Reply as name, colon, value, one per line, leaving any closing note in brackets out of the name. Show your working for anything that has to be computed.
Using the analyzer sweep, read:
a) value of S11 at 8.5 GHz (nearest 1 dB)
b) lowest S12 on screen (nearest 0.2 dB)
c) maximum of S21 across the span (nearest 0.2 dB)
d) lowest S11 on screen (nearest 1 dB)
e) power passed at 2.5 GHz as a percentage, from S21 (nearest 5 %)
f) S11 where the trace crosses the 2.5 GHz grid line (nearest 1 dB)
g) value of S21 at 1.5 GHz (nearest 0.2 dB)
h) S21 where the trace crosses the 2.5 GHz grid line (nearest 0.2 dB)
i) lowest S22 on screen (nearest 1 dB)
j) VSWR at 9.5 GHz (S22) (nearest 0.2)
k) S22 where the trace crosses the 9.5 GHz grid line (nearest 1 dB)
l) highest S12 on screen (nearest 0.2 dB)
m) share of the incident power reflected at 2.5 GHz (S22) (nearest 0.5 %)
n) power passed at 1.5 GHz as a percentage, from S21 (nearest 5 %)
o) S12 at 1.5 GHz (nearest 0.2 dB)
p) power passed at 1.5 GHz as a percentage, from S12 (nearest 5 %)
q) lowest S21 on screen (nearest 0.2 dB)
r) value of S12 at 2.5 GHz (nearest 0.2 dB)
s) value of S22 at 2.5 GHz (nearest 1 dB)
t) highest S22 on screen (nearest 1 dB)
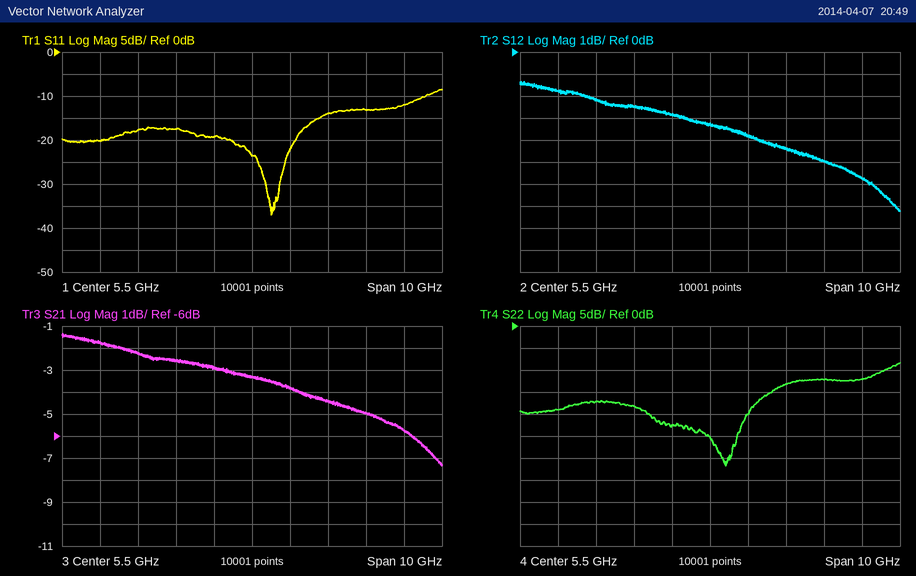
value of S11 at 8.5 GHz: -13 dB
lowest S12 on screen: -7.2 dB
maximum of S21 across the span: -1.4 dB
lowest S11 on screen: -37 dB
power passed at 2.5 GHz as a percentage, from S21: 10^(-2.2/10) ≈ 60 %
S11 where the trace crosses the 2.5 GHz grid line: -18 dB
value of S21 at 1.5 GHz: -1.8 dB
S21 where the trace crosses the 2.5 GHz grid line: -2.2 dB
lowest S22 on screen: -32 dB
VSWR at 9.5 GHz (S22): |Γ| = 10^(-12/20) = 0.2512; VSWR = (1 + 0.2512)/(1 − 0.2512) ≈ 1.67, so 1.6 to the nearest 0.2
S22 where the trace crosses the 9.5 GHz grid line: -12 dB
highest S12 on screen: -1.4 dB
share of the incident power reflected at 2.5 GHz (S22): 10^(-17/10) ≈ 2.0 %
power passed at 1.5 GHz as a percentage, from S21: 10^(-1.8/10) ≈ 66.1 %, so 65 % to the nearest 5 %
S12 at 1.5 GHz: -1.8 dB
power passed at 1.5 GHz as a percentage, from S12: 10^(-1.8/10) ≈ 66.1 %, so 65 % to the nearest 5 %
lowest S21 on screen: -7.4 dB
value of S12 at 2.5 GHz: -2.2 dB
value of S22 at 2.5 GHz: -17 dB
highest S22 on screen: -8 dB
